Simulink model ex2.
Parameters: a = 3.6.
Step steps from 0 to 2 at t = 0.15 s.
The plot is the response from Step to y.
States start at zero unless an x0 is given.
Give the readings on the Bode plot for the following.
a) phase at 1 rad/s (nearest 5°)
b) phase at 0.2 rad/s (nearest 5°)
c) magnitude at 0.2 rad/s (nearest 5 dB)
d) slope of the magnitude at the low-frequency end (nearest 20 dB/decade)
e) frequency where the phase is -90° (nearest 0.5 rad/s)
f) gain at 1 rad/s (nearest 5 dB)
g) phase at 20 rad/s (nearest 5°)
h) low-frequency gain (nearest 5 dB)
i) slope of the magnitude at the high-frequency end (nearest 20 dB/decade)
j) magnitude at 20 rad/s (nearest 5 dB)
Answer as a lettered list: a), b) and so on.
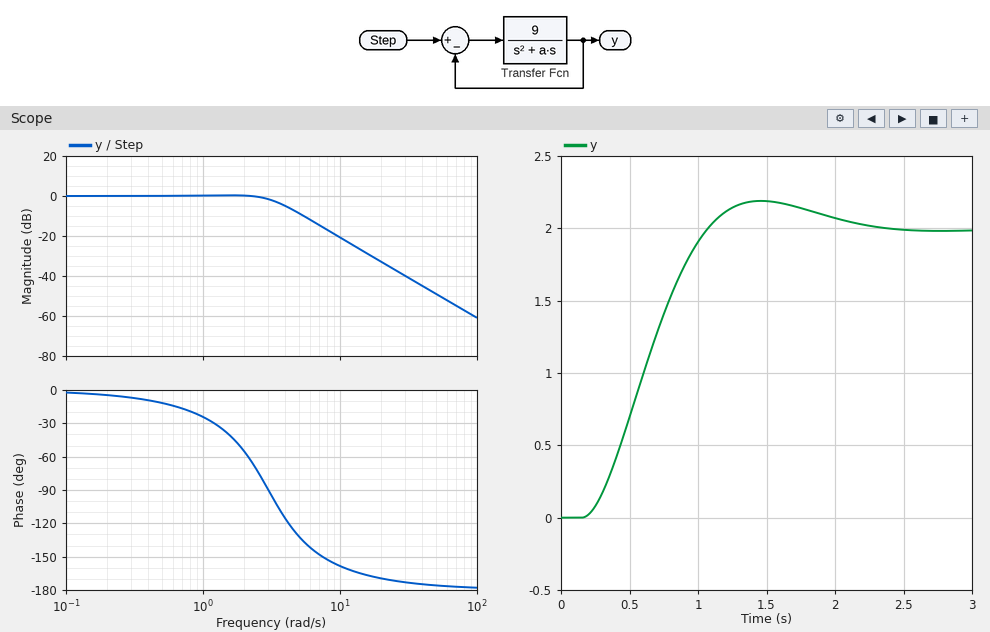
a) -25°
b) -5°
c) 0 dB
d) 0 dB/decade
e) 3.0 rad/s
f) 0 dB
g) -170°
h) 0 dB
i) -40 dB/decade
j) -35 dB
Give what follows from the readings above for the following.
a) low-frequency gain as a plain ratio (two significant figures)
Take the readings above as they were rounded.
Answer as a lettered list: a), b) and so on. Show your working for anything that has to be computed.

a) 10^(0 / 20) = 1.0
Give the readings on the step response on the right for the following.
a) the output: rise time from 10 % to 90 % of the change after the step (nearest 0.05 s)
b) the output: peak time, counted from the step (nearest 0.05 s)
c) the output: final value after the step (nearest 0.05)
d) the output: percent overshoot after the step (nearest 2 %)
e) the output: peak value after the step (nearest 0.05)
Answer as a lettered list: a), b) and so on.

a) 0.60 s
b) 1.30 s
c) 2.00
d) 10 %
e) 2.20
